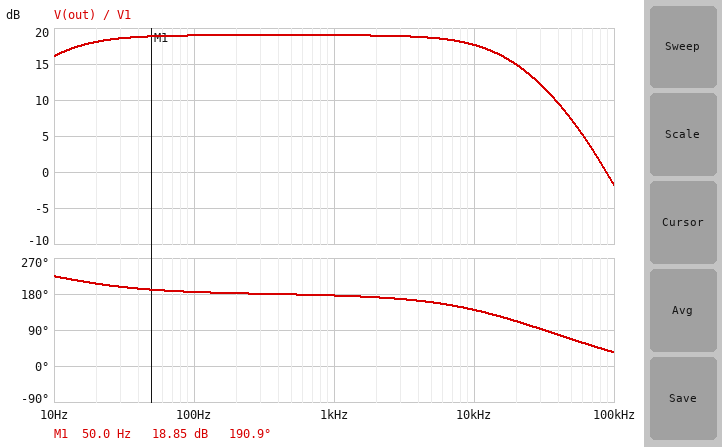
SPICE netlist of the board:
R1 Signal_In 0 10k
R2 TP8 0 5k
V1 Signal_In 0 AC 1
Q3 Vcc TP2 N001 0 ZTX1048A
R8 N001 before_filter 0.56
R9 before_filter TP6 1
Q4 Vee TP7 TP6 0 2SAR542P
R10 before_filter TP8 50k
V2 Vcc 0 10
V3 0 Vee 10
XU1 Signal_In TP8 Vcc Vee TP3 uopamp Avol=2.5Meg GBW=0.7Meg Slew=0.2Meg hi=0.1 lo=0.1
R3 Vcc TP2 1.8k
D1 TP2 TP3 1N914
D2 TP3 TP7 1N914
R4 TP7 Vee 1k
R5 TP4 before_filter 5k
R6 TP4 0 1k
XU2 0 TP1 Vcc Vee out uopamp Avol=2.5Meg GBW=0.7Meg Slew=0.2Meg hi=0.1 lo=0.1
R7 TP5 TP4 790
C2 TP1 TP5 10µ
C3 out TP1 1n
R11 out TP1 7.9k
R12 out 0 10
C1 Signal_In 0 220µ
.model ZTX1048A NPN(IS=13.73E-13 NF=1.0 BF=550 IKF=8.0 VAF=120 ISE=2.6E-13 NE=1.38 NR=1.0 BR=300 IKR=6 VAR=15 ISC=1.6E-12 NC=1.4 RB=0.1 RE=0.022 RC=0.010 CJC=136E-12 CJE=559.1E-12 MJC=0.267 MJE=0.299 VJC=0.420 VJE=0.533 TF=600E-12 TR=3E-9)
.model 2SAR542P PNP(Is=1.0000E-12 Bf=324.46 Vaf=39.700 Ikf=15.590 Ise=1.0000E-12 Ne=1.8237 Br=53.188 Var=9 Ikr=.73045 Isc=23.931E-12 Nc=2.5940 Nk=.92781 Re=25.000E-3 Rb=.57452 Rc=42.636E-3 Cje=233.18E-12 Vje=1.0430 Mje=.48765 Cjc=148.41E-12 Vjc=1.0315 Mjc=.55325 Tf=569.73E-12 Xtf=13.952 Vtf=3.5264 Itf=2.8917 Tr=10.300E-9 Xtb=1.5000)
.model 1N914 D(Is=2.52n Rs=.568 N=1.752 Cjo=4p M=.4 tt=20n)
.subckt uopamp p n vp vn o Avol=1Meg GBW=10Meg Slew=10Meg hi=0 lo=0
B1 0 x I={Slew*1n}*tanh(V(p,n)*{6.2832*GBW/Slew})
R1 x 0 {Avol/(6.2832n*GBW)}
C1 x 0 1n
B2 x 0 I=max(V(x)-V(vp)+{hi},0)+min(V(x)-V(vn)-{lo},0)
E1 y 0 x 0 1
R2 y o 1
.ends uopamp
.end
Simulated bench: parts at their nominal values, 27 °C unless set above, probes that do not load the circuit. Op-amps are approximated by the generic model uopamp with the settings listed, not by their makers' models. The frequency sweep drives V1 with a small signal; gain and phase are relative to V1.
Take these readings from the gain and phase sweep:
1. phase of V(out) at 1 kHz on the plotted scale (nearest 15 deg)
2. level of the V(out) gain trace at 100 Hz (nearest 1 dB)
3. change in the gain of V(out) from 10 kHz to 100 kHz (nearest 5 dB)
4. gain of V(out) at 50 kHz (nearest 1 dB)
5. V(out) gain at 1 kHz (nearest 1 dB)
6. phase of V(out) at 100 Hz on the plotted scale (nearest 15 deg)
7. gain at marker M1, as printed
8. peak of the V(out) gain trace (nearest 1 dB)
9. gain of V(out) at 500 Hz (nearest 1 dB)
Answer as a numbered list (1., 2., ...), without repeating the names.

1. 180 deg
2. 19 dB
3. -20 dB
4. 7 dB
5. 19 dB
6. 180 deg
7. 18.85 dB
8. 19 dB
9. 19 dB
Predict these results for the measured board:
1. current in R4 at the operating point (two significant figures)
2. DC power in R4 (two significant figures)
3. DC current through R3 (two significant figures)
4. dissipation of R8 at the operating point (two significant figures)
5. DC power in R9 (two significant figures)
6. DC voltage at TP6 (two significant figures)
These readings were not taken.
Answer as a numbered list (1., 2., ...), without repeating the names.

1. 9.3 mA
2. 87 mW
3. 5.2 mA
4. 1.6 mW
5. 2.8 mW
6. -53 mV
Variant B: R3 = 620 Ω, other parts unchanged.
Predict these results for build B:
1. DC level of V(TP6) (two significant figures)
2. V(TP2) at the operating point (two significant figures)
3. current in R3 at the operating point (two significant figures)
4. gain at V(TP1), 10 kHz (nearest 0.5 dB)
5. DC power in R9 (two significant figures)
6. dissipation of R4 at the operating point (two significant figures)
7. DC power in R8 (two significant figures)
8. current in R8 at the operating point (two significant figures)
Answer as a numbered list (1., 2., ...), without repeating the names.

1. -75 mV
2. 680 mV
3. 15 mA
4. -18.5 dB
5. 5.7 mW
6. 86 mW
7. 3.2 mW
8. 75 mA
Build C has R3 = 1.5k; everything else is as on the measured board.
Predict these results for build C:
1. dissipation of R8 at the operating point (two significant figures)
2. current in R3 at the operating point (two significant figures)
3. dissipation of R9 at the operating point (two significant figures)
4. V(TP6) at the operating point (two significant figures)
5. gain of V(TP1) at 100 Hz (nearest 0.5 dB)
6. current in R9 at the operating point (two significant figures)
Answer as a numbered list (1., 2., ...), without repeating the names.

1. 1.8 mW
2. 6.2 mA
3. 3.2 mW
4. -57 mV
5. -57.0 dB
6. 57 mA
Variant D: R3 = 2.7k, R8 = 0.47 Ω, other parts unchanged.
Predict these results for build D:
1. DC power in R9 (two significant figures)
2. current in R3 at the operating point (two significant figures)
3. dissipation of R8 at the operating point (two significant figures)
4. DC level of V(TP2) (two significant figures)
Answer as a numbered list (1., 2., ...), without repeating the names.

1. 2.3 mW
2. 3.5 mA
3. 1.1 mW
4. 650 mV
